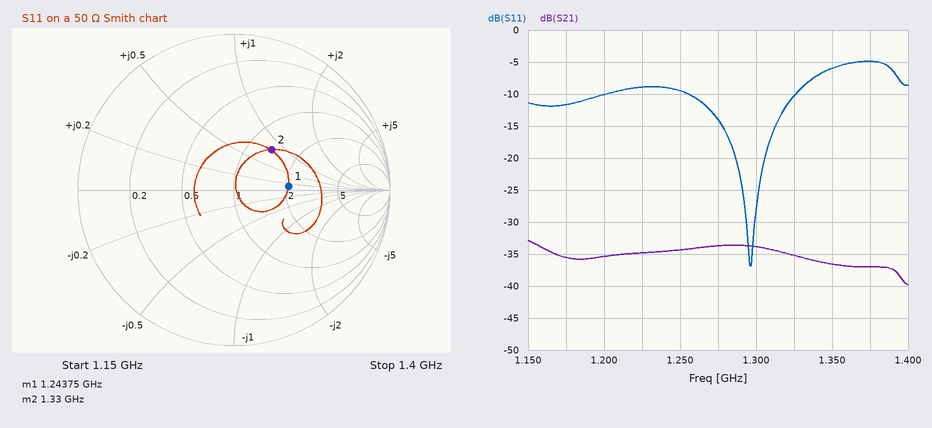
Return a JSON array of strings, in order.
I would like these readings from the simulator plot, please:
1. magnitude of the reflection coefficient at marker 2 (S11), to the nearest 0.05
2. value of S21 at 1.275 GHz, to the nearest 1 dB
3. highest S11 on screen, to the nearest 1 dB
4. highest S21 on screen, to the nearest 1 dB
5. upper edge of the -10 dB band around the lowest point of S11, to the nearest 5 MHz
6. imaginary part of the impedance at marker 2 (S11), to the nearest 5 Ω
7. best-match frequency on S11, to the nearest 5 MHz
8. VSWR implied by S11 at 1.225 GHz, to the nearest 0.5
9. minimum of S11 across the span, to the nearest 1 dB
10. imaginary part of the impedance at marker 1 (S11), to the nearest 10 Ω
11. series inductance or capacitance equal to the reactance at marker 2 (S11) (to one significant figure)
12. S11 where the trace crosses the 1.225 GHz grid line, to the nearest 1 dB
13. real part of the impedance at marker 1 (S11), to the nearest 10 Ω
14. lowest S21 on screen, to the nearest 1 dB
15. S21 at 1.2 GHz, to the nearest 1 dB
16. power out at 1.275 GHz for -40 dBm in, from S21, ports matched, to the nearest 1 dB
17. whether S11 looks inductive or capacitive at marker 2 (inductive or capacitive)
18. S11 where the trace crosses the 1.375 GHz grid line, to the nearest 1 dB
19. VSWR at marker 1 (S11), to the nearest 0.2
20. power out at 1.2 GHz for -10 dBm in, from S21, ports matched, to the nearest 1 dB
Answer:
["0.35", "-34 dB", "-5 dB", "-33 dB", "1.325 GHz", "+40 Ω", "1.295 GHz", "2.0", "-37 dB", "+10 Ω", "5 nH", "-9 dB", "100 Ω", "-40 dB", "-35 dB", "-74 dBm", "inductive", "-5 dB", "2.0", "-45 dBm"]
